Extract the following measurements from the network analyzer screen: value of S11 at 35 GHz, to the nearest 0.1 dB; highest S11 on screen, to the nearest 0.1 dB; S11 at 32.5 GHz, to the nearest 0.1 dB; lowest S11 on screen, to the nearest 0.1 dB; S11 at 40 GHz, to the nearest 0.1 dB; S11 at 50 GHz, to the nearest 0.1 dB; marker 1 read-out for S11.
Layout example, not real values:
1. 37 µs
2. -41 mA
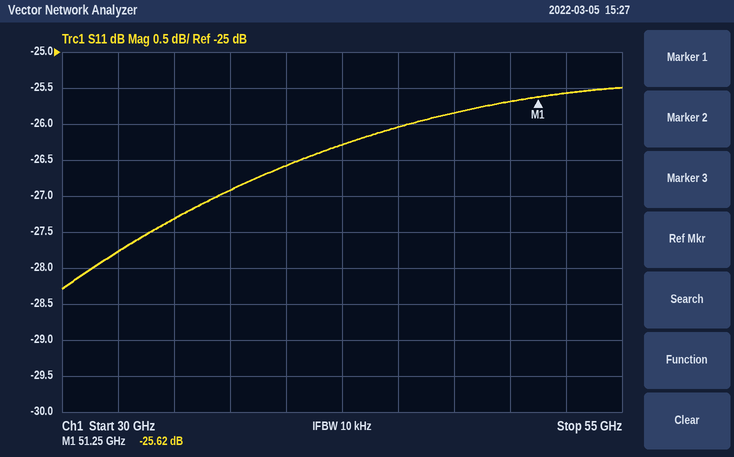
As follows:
1. -27.3 dB
2. -25.5 dB
3. -27.8 dB
4. -28.3 dB
5. -26.6 dB
6. -25.7 dB
7. -25.62 dB
